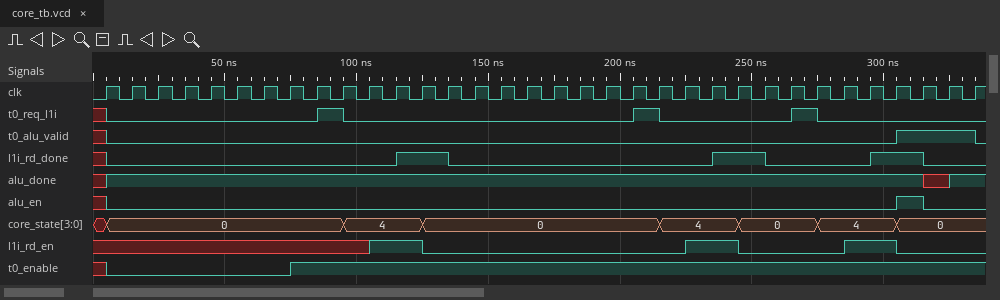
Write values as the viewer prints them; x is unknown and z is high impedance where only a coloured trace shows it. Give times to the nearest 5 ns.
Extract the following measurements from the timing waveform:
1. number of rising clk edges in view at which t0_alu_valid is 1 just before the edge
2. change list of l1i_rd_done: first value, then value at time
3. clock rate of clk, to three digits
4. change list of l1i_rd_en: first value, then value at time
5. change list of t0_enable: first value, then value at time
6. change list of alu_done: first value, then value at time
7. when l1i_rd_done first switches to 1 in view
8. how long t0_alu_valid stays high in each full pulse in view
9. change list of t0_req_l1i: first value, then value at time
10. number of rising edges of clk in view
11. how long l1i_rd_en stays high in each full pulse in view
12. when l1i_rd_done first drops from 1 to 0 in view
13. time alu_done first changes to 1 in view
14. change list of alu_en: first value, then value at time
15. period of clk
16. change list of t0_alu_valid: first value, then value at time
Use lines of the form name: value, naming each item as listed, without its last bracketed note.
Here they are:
number of rising clk edges in view at which t0_alu_valid is 1 just before the edge: 3
change list of l1i_rd_done: first value, then value at time: x, 0 at 5 ns, 1 at 115 ns, 0 at 135 ns, 1 at 235 ns, 0 at 255 ns, 1 at 295 ns, 0 at 315 ns
clock rate of clk, to three digits: 100 MHz
change list of l1i_rd_en: first value, then value at time: x, 1 at 105 ns, 0 at 125 ns, 1 at 225 ns, 0 at 245 ns, 1 at 285 ns, 0 at 305 ns
change list of t0_enable: first value, then value at time: x, 0 at 5 ns, 1 at 75 ns
change list of alu_done: first value, then value at time: x, 1 at 5 ns, x at 315 ns, 1 at 325 ns
when l1i_rd_done first switches to 1 in view: 115 ns
how long t0_alu_valid stays high in each full pulse in view: 30 ns
change list of t0_req_l1i: first value, then value at time: x, 0 at 5 ns, 1 at 85 ns, 0 at 95 ns, 1 at 205 ns, 0 at 215 ns, 1 at 265 ns, 0 at 275 ns
number of rising edges of clk in view: 34
how long l1i_rd_en stays high in each full pulse in view: 20 ns, 20 ns
when l1i_rd_done first drops from 1 to 0 in view: 135 ns
time alu_done first changes to 1 in view: 5 ns
change list of alu_en: first value, then value at time: x, 0 at 5 ns, 1 at 305 ns, 0 at 315 ns
period of clk: 10 ns
change list of t0_alu_valid: first value, then value at time: x, 0 at 5 ns, 1 at 305 ns, 0 at 335 ns
